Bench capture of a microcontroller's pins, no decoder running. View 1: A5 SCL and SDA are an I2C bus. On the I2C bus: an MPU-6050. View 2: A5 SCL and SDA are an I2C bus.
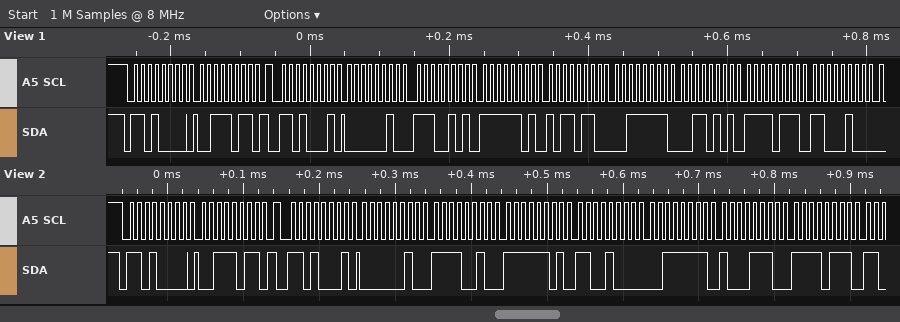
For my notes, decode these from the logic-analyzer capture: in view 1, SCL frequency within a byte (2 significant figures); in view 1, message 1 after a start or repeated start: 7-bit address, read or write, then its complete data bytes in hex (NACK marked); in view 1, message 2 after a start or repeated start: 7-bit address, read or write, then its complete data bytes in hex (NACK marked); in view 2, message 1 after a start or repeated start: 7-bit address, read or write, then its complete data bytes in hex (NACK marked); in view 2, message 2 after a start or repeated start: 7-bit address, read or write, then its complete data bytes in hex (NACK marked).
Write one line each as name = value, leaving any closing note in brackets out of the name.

in view 1, SCL frequency within a byte = 100 kHz
in view 1, message 1 after a start or repeated start: 7-bit address, read or write, then its complete data bytes in hex = 0x68 write: 3B
in view 1, message 2 after a start or repeated start: 7-bit address, read or write, then its complete data bytes in hex = 0x68 read: 02 E5 FD B6 3F 35 F7 C4
in view 2, message 1 after a start or repeated start: 7-bit address, read or write, then its complete data bytes in hex = 0x68 write: 3B
in view 2, message 2 after a start or repeated start: 7-bit address, read or write, then its complete data bytes in hex = 0x68 read: 02 F2 FD C8 3F 8E F7
